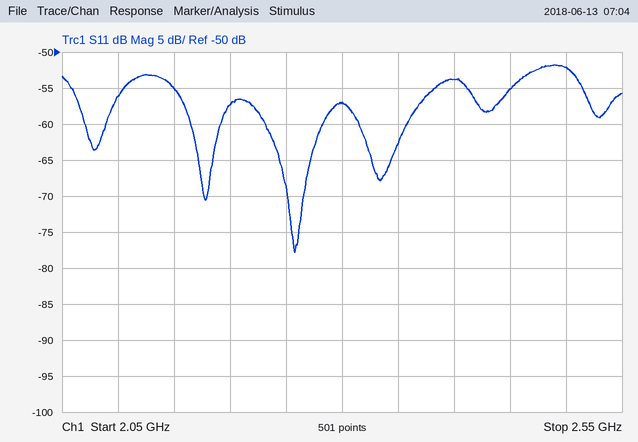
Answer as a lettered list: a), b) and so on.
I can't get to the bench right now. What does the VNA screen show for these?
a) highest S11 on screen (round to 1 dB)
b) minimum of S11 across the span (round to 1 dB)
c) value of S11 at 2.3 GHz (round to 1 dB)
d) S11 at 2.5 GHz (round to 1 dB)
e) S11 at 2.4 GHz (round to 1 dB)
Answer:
a) -52 dB
b) -78 dB
c) -57 dB
d) -52 dB
e) -54 dB
